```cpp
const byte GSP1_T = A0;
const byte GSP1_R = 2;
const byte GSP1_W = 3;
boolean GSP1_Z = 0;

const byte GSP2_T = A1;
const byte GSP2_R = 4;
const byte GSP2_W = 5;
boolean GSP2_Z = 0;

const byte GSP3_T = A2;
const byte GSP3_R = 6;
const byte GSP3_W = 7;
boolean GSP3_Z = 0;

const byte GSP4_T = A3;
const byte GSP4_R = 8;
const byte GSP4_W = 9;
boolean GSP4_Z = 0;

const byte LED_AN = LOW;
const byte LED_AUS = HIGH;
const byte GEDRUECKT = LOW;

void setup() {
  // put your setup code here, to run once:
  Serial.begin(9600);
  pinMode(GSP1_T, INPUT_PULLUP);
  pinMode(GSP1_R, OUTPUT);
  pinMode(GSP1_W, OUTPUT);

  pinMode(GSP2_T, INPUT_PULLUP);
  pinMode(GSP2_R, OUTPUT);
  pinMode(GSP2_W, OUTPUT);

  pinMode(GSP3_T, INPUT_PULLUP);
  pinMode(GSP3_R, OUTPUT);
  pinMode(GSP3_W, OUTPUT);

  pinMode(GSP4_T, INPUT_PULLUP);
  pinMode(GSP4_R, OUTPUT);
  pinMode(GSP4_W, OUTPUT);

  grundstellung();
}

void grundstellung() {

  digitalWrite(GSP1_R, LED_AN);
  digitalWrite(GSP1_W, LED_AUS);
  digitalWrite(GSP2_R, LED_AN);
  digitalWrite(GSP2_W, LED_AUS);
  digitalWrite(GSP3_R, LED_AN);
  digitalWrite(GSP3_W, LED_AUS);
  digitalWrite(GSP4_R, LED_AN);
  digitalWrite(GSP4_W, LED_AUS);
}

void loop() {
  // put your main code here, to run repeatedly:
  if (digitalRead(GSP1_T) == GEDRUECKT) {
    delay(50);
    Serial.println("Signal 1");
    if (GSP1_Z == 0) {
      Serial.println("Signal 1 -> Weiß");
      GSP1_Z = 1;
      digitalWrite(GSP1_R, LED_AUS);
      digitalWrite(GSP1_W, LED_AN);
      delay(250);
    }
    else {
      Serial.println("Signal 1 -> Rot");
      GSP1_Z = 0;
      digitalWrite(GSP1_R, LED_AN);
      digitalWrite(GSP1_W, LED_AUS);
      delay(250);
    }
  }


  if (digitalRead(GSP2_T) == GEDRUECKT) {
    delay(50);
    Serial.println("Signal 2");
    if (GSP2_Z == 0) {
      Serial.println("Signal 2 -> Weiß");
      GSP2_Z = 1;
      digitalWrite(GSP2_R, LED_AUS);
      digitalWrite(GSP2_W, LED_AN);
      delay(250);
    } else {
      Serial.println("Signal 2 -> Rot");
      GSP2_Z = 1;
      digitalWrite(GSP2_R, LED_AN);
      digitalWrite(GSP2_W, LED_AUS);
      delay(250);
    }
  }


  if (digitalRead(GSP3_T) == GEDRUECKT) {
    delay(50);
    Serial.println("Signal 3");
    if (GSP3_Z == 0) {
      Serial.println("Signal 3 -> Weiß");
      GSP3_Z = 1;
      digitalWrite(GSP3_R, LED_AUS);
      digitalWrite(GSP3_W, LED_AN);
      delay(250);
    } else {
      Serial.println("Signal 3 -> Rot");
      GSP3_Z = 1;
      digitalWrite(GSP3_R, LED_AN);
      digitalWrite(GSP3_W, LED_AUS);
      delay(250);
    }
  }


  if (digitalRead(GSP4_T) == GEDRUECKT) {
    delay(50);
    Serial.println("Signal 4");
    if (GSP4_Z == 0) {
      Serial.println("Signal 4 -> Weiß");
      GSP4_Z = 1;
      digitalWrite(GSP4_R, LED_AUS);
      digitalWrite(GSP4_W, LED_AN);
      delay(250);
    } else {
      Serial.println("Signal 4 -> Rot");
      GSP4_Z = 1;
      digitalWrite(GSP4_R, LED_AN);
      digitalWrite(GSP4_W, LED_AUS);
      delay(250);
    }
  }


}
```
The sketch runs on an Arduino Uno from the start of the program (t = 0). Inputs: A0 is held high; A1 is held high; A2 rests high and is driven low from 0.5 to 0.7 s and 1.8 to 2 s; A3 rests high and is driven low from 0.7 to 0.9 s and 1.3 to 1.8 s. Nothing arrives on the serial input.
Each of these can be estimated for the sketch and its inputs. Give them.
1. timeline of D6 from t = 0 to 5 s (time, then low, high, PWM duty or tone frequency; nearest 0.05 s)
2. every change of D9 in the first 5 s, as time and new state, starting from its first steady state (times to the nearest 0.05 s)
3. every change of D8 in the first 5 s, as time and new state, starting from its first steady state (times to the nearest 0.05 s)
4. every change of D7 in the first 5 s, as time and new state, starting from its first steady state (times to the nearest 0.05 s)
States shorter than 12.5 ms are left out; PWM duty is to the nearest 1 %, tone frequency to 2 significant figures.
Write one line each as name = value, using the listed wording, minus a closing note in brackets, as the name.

timeline of D6 from t = 0 to 5 s = 0 s low; 0.55 s high; 1.95 s low
every change of D9 in the first 5 s, as time and new state, starting from its first steady state = 0 s high; 0.85 s low; 1.35 s high
every change of D8 in the first 5 s, as time and new state, starting from its first steady state = 0 s low; 0.85 s high; 1.35 s low
every change of D7 in the first 5 s, as time and new state, starting from its first steady state = 0 s high; 0.55 s low; 1.95 s high
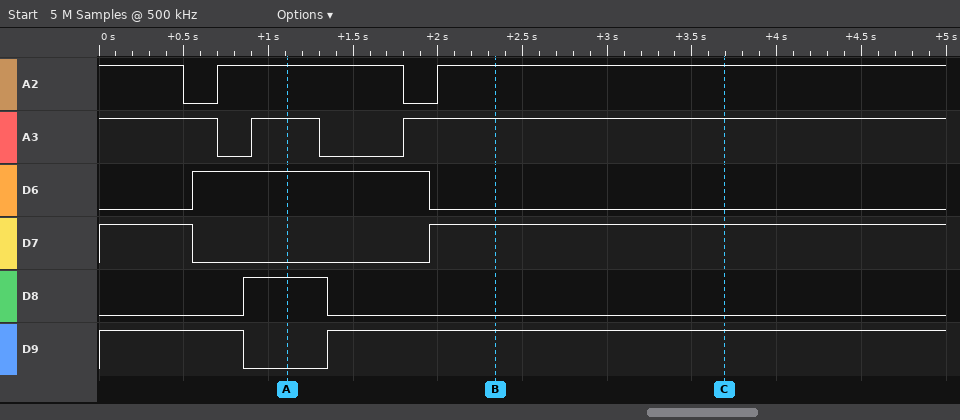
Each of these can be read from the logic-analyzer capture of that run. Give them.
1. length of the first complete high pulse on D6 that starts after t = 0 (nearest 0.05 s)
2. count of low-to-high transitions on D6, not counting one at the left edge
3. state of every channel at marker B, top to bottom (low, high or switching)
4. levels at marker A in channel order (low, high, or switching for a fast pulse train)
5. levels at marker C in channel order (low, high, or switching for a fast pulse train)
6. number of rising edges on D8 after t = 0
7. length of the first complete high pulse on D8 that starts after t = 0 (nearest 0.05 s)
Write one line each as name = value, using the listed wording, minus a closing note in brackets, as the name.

length of the first complete high pulse on D6 that starts after t = 0 = 1.40 s
count of low-to-high transitions on D6, not counting one at the left edge = 1
state of every channel at marker B, top to bottom = A2 high, A3 high, D6 low, D7 high, D8 low, D9 high
levels at marker A in channel order = A2 high, A3 high, D6 high, D7 low, D8 high, D9 low
levels at marker C in channel order = A2 high, A3 high, D6 low, D7 high, D8 low, D9 high
number of rising edges on D8 after t = 0 = 1
length of the first complete high pulse on D8 that starts after t = 0 = 0.50 s
